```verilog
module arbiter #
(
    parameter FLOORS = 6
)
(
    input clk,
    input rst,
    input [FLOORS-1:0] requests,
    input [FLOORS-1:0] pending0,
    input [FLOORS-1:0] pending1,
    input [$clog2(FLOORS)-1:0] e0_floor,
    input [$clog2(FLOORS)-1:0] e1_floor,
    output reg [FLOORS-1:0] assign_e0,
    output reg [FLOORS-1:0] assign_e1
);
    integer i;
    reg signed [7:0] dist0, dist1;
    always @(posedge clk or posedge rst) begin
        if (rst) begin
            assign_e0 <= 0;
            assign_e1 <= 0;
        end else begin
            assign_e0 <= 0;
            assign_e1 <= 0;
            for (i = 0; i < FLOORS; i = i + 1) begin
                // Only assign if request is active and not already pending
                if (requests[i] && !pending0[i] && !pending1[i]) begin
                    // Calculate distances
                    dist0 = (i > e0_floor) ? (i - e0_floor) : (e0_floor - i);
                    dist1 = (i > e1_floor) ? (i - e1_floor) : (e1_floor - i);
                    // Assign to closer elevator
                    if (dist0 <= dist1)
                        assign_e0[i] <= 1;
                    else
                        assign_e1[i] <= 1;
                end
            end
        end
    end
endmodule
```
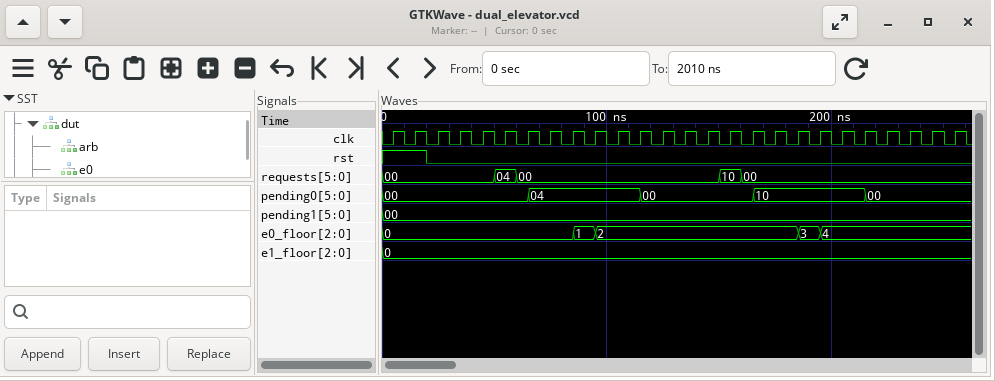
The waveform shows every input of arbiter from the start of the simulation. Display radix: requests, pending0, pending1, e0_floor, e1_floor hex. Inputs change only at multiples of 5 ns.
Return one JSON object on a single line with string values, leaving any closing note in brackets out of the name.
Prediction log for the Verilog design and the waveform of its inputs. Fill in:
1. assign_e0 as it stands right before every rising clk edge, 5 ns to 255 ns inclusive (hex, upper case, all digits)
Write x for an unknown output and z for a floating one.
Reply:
{"assign_e0 as it stands right before every rising clk edge, 5 ns to 255 ns inclusive": "00, 00, 00, 00, 00, 00, 04, 00, 00, 00, 00, 00, 00, 00, 00, 00, 10, 00, 00, 00, 00, 00, 00, 00, 00, 00"}
